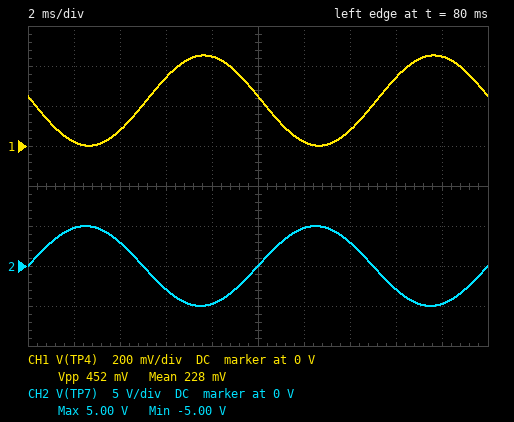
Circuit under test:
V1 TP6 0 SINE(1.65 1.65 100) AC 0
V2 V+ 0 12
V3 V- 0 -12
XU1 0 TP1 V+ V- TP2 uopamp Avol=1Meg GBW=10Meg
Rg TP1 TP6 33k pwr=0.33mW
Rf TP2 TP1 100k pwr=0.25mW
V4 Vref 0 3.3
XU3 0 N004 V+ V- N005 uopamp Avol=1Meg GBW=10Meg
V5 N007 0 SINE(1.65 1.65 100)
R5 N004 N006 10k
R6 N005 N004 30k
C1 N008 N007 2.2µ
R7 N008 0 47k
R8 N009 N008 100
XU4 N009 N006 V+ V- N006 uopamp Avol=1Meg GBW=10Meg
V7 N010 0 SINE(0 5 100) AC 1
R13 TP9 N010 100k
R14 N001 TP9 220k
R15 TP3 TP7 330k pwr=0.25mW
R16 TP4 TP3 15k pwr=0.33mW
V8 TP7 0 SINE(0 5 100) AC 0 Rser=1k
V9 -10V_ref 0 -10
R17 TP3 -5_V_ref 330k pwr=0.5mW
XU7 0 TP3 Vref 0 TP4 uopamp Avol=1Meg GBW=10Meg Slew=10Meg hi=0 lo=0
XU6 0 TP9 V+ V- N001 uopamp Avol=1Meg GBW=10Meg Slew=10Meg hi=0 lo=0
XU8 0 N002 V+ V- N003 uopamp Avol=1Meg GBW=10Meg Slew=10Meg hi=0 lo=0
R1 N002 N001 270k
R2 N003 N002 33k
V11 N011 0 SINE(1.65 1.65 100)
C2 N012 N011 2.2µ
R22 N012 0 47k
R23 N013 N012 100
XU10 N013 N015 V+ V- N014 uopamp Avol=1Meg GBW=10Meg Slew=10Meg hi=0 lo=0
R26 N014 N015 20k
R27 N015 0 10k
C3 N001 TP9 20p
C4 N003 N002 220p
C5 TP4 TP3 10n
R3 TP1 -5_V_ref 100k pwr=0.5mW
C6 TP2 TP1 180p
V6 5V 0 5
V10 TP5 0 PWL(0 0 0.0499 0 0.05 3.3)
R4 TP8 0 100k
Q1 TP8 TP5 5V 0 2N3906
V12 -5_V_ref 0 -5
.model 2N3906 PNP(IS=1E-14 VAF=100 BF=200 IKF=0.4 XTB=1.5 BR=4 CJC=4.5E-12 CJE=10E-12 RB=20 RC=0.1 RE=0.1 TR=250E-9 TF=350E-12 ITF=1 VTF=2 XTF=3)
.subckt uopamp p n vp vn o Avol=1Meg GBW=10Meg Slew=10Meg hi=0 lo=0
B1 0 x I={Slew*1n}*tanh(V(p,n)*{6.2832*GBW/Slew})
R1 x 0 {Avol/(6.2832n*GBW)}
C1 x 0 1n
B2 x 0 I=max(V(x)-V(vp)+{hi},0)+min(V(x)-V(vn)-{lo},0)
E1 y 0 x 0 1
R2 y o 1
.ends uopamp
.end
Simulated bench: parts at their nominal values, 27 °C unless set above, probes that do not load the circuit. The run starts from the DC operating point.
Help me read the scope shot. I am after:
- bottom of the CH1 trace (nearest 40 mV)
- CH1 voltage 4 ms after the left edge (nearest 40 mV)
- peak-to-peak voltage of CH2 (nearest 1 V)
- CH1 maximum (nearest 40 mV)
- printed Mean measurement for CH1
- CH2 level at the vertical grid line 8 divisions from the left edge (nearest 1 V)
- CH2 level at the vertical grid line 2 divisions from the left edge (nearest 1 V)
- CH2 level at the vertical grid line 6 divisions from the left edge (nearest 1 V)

0 V
80 mV
10 V
440 mV
228 mV
-3 V
3 V
5 V
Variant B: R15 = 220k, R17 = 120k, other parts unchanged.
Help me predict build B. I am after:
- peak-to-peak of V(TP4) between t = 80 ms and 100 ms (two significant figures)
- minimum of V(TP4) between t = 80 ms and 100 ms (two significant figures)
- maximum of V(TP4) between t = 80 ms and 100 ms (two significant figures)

680 mV
290 mV
960 mV
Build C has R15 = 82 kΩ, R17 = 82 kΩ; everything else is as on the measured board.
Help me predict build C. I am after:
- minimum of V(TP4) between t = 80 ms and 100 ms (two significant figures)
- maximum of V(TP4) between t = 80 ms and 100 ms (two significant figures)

15 mV
1.8 V
